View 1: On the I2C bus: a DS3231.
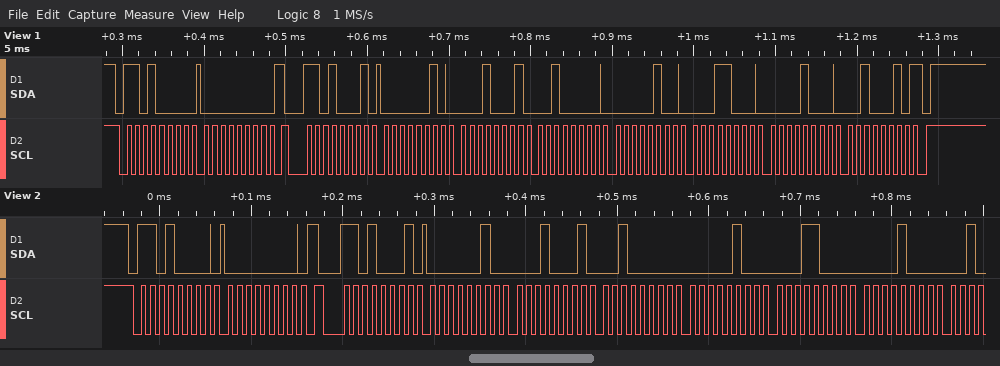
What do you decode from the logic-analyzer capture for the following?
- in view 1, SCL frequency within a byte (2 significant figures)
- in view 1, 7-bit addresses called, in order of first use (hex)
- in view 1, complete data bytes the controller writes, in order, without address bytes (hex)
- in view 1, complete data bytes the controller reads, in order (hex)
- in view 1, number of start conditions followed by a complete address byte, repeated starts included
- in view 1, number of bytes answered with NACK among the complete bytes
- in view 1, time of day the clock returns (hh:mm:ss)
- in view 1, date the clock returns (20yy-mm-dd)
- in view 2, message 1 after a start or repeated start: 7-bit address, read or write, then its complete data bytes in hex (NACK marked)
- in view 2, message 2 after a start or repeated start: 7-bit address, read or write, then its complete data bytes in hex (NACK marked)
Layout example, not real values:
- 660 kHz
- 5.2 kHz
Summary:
- 100 kHz
- 0x68
- 00
- 02 11 20 04 18 08 22
- 2
- 1
- 20:11:02
- 2022-08-18
- 0x68 write: 00
- 0x68 read: 02 11 20 04 18 08
